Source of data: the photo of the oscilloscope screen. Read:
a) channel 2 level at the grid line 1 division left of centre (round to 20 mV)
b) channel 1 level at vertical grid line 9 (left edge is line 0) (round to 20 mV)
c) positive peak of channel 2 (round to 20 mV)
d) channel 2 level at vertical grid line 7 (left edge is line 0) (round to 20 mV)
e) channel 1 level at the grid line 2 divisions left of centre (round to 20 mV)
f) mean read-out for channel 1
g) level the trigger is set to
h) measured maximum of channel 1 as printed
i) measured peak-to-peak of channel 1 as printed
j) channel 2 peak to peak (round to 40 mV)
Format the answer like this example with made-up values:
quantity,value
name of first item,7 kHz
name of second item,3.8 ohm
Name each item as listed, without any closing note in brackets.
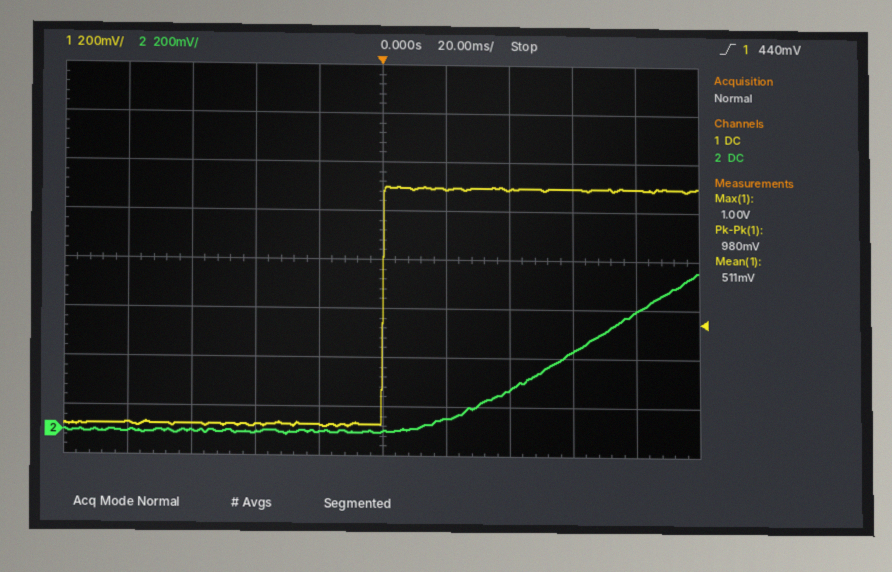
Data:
quantity,value
channel 2 level at the grid line 1 division left of centre,0 mV
channel 1 level at vertical grid line 9 (left edge is line 0),1.00 V
positive peak of channel 2,660 mV
channel 2 level at vertical grid line 7 (left edge is line 0),180 mV
channel 1 level at the grid line 2 divisions left of centre,20 mV
mean read-out for channel 1,511 mV
level the trigger is set to,440 mV
measured maximum of channel 1 as printed,1.00 V
measured peak-to-peak of channel 1 as printed,980 mV
channel 2 peak to peak,680 mV
